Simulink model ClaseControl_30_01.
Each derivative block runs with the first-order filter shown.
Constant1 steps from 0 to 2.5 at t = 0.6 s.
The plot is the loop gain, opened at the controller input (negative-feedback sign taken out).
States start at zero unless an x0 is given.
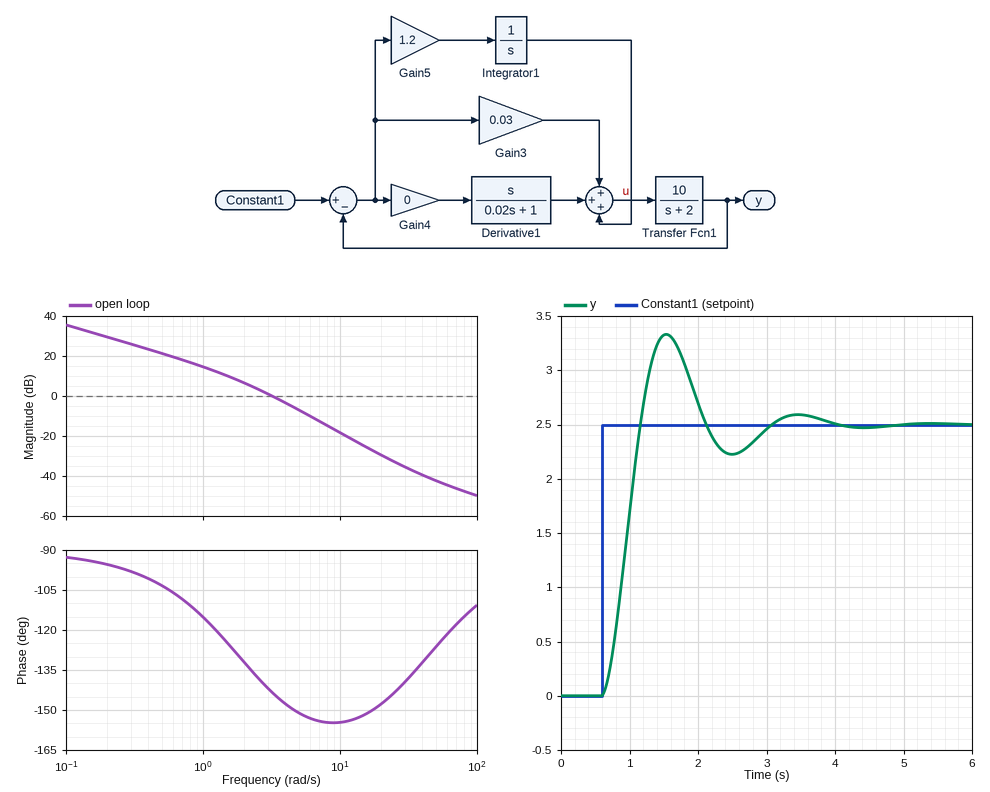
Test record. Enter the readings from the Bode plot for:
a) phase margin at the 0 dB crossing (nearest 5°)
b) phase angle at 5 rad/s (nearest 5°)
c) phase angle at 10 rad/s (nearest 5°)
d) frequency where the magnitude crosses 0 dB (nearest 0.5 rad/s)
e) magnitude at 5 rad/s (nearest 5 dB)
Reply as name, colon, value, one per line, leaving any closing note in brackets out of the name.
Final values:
phase margin at the 0 dB crossing: 35°
phase angle at 5 rad/s: -150°
phase angle at 10 rad/s: -155°
frequency where the magnitude crosses 0 dB: 3.0 rad/s
magnitude at 5 rad/s: -5 dB
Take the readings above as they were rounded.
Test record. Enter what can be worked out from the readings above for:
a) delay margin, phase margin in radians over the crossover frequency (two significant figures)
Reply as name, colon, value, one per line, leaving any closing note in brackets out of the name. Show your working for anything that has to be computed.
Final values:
delay margin, phase margin in radians over the crossover frequency: 35 × π / 180 / 3 = 0.20 s
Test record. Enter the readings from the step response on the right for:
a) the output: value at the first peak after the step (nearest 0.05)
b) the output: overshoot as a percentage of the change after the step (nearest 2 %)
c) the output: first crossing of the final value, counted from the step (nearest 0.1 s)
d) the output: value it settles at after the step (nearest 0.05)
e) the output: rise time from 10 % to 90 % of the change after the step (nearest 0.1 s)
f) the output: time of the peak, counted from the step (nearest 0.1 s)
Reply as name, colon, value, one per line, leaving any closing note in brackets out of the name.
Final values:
the output: value at the first peak after the step: 3.35
the output: overshoot as a percentage of the change after the step: 34 %
the output: first crossing of the final value, counted from the step: 0.6 s
the output: value it settles at after the step: 2.50
the output: rise time from 10 % to 90 % of the change after the step: 0.4 s
the output: time of the peak, counted from the step: 0.9 s
